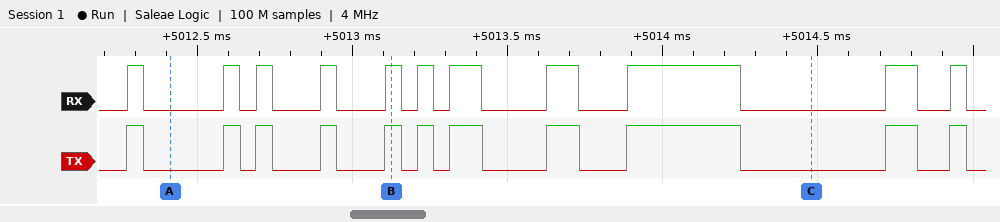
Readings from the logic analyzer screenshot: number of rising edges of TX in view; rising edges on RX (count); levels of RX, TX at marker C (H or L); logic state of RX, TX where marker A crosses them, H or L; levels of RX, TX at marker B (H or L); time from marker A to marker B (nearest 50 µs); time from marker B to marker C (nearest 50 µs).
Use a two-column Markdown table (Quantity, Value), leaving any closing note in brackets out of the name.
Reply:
| Quantity | Value |
|---|---|
| number of rising edges of TX in view | 11 |
| rising edges on RX | 11 |
| levels of RX, TX at marker C | RX=L, TX=L |
| logic state of RX, TX where marker A crosses them, H or L | RX=L, TX=L |
| levels of RX, TX at marker B | RX=H, TX=H |
| time from marker A to marker B | 700 µs |
| time from marker B to marker C | 1350 µs |
